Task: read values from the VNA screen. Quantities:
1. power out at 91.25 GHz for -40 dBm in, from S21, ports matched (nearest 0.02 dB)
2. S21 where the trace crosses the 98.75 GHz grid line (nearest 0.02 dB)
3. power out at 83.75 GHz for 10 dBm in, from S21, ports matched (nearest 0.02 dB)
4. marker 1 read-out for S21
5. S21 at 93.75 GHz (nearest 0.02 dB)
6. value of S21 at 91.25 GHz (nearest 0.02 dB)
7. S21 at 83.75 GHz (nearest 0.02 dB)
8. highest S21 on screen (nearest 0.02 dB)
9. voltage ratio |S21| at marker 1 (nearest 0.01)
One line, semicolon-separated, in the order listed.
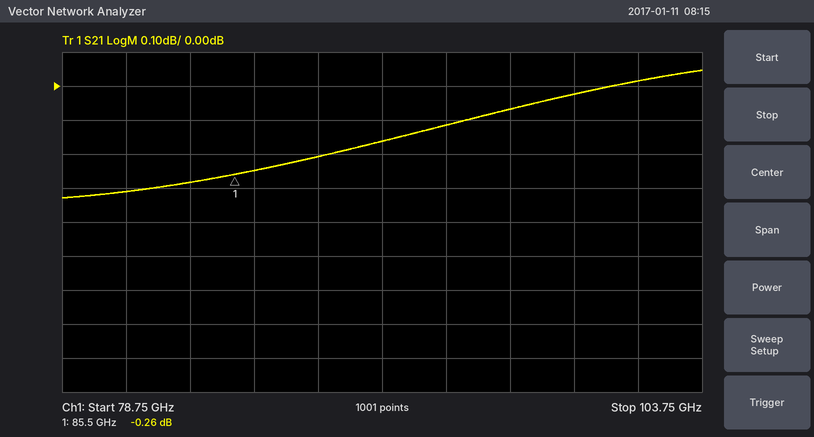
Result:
-40.16 dBm; -0.02 dB; 9.72 dBm; -0.26 dB; -0.12 dB; -0.16 dB; -0.28 dB; 0.04 dB; 0.97
